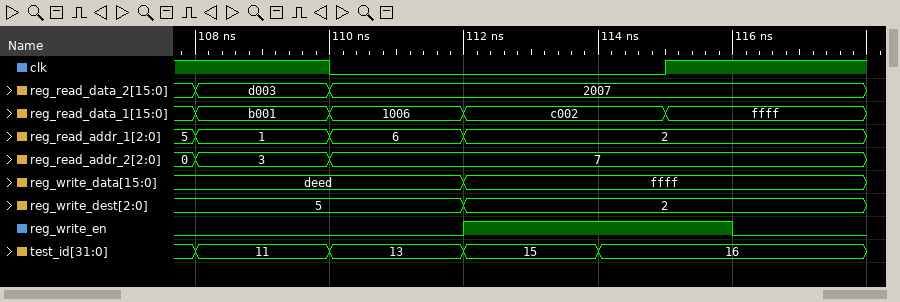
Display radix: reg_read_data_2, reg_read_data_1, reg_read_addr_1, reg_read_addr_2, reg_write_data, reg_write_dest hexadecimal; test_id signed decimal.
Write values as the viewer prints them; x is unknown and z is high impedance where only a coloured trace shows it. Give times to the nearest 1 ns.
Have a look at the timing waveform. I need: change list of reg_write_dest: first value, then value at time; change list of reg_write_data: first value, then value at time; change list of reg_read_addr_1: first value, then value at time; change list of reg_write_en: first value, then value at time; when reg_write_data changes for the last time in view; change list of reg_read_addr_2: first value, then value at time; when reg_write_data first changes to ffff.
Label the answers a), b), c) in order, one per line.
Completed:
a) 5, 2 at 112 ns
b) deed, ffff at 112 ns
c) 5, 1 at 108 ns, 6 at 110 ns, 2 at 112 ns
d) 0, 1 at 112 ns, 0 at 116 ns
e) 112 ns
f) 0, 3 at 108 ns, 7 at 110 ns
g) 112 ns
